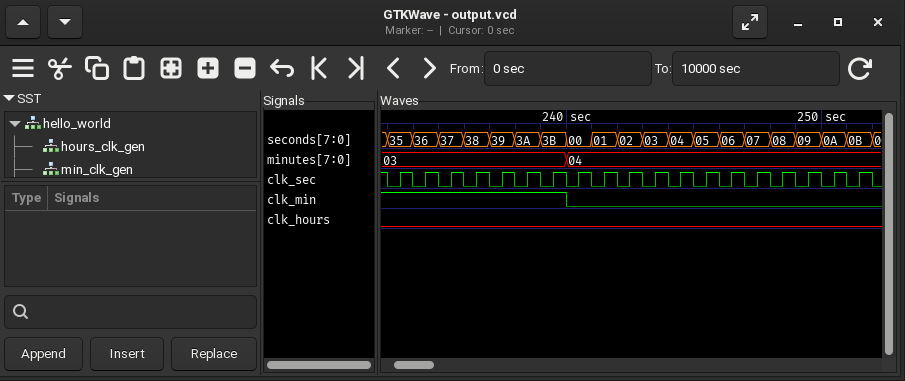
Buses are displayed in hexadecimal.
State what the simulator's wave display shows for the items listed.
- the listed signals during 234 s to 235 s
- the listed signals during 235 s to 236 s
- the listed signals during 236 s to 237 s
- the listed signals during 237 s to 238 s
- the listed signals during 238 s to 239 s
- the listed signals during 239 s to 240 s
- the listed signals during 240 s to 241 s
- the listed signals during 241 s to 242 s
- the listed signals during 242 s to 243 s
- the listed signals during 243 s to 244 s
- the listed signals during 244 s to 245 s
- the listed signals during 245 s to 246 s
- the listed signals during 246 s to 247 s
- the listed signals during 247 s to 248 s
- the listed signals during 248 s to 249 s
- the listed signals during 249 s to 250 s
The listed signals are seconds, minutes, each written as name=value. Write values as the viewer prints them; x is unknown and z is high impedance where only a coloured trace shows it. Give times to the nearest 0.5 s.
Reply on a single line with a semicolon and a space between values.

seconds=36, minutes=03; seconds=37, minutes=03; seconds=38, minutes=03; seconds=39, minutes=03; seconds=3A, minutes=03; seconds=3B, minutes=03; seconds=00, minutes=04; seconds=01, minutes=04; seconds=02, minutes=04; seconds=03, minutes=04; seconds=04, minutes=04; seconds=05, minutes=04; seconds=06, minutes=04; seconds=07, minutes=04; seconds=08, minutes=04; seconds=09, minutes=04
